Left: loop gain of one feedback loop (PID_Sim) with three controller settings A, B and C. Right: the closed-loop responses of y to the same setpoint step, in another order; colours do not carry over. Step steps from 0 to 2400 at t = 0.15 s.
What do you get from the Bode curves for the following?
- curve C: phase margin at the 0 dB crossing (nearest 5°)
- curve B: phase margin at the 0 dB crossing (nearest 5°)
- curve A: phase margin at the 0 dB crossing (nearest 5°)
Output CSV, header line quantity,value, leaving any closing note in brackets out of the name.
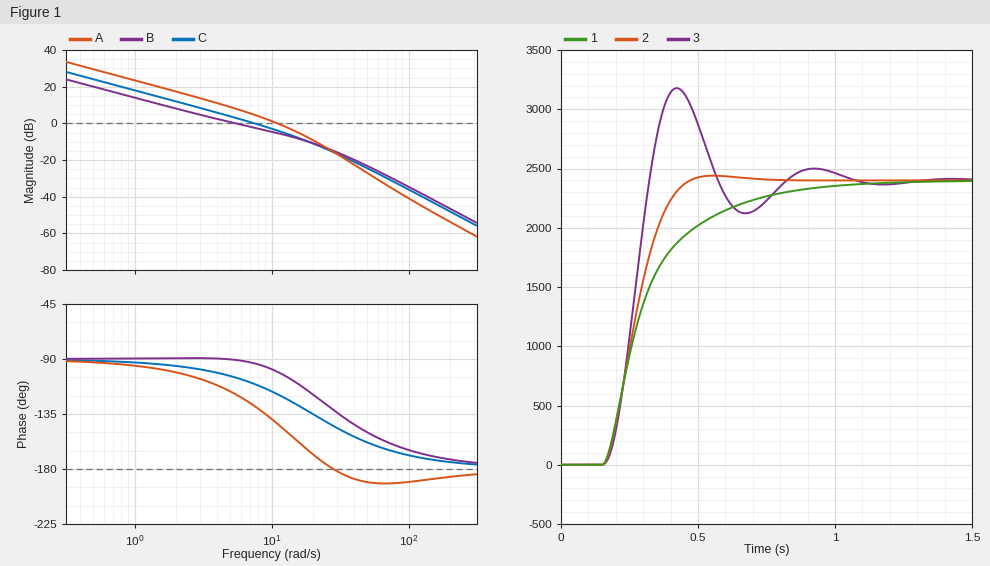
quantity,value
curve C: phase margin at the 0 dB crossing,70°
curve B: phase margin at the 0 dB crossing,90°
curve A: phase margin at the 0 dB crossing,35°
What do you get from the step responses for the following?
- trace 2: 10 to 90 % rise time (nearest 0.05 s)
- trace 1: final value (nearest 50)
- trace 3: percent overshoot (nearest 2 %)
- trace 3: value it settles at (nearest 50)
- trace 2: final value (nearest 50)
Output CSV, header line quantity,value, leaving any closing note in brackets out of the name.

quantity,value
trace 2: 10 to 90 % rise time,0.20 s
trace 1: final value,2400
trace 3: percent overshoot,32 %
trace 3: value it settles at,2400
trace 2: final value,2400
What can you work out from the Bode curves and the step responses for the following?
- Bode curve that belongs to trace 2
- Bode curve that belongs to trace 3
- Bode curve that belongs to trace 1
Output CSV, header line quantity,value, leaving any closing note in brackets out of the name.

quantity,value
Bode curve that belongs to trace 2,C
Bode curve that belongs to trace 3,A
Bode curve that belongs to trace 1,B
